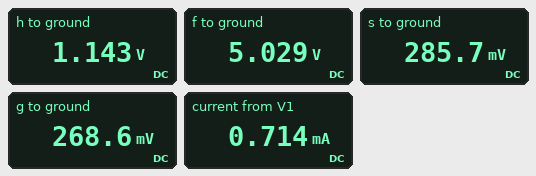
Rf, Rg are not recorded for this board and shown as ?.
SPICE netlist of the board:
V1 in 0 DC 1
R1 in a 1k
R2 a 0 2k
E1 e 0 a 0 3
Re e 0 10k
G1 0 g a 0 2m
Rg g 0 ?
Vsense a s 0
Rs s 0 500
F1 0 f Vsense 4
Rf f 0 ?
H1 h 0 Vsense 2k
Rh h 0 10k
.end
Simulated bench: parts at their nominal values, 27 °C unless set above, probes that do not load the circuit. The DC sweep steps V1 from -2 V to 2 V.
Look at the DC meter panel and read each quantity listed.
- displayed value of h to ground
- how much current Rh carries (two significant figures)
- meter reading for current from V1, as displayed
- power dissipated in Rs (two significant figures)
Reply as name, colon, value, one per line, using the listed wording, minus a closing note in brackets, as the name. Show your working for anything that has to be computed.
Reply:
displayed value of h to ground: 1.143 V
how much current Rh carries: (1.143 V) / 10 kΩ = 110 µA
meter reading for current from V1, as displayed: 0.714 mA
power dissipated in Rs: (285.7 mV)^2 / 500 Ω = 160 µW
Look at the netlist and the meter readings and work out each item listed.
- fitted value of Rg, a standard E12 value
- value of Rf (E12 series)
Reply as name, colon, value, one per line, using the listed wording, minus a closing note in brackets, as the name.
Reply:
fitted value of Rg, a standard E12 value: 470 Ω
value of Rf: 2.2 kΩ
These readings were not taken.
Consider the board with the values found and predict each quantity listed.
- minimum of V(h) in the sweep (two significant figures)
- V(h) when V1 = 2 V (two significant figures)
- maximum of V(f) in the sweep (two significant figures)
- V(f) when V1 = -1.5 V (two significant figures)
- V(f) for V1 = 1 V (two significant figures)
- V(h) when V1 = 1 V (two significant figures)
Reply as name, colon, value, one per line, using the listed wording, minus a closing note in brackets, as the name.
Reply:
minimum of V(h) in the sweep: -2.3 V
V(h) when V1 = 2 V: 2.3 V
maximum of V(f) in the sweep: 10 V
V(f) when V1 = -1.5 V: -7.5 V
V(f) for V1 = 1 V: 5.0 V
V(h) when V1 = 1 V: 1.1 V
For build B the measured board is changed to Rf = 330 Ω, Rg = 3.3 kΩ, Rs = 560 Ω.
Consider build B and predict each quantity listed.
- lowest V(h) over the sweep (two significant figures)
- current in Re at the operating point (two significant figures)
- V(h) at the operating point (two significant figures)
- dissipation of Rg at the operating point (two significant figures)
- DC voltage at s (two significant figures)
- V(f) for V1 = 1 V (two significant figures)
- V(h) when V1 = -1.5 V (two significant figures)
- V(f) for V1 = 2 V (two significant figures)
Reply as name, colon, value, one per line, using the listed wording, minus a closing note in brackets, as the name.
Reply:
lowest V(h) over the sweep: -2.2 V
current in Re at the operating point: 91 µA
V(h) at the operating point: 1.1 V
dissipation of Rg at the operating point: 1.2 mW
DC voltage at s: 300 mV
V(f) for V1 = 1 V: 720 mV
V(h) when V1 = -1.5 V: -1.6 V
V(f) for V1 = 2 V: 1.4 V
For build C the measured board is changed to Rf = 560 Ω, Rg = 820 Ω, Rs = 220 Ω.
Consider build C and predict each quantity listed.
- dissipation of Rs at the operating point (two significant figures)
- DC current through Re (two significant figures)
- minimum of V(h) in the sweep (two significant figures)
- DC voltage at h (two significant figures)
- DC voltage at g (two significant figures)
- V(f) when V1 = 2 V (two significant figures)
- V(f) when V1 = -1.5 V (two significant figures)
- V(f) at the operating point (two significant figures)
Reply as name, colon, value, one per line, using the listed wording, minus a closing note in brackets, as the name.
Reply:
dissipation of Rs at the operating point: 120 µW
DC current through Re: 50 µA
minimum of V(h) in the sweep: -3.0 V
DC voltage at h: 1.5 V
DC voltage at g: 270 mV
V(f) when V1 = 2 V: 3.4 V
V(f) when V1 = -1.5 V: -2.5 V
V(f) at the operating point: 1.7 V
